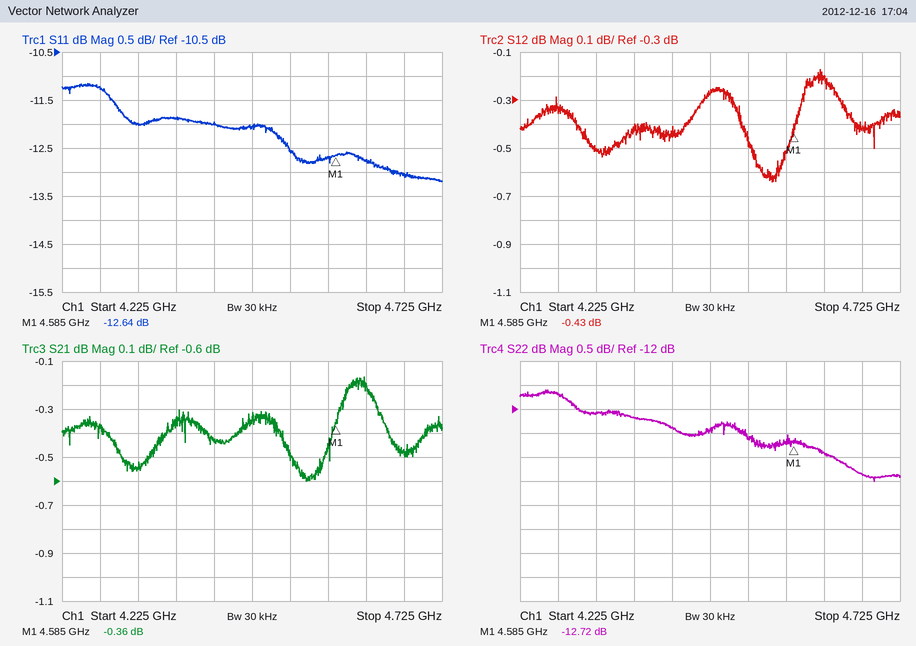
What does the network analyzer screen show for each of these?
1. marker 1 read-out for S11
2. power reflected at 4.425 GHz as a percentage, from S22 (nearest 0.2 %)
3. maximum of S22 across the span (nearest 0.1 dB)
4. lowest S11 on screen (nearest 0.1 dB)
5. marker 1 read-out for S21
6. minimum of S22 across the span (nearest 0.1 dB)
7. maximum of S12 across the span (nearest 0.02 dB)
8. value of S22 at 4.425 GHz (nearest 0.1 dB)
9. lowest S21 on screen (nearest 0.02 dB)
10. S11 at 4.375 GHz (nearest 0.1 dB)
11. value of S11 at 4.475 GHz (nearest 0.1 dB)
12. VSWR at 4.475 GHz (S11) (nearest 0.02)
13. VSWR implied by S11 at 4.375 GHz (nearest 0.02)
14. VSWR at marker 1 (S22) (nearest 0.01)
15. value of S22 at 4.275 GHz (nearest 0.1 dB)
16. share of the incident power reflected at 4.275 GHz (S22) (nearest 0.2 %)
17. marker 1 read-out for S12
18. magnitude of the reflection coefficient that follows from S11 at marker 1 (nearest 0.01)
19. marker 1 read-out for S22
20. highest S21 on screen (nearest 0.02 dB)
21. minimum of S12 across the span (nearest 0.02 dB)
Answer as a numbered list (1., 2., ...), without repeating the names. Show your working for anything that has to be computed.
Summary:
1. -12.64 dB
2. 10^(-12.4/10) ≈ 5.8 %
3. -11.6 dB
4. -13.2 dB
5. -0.36 dB
6. -13.5 dB
7. -0.18 dB
8. -12.4 dB
9. -0.60 dB
10. -11.9 dB
11. -12.1 dB
12. |Γ| = 10^(-12.1/20) = 0.2483; VSWR = (1 + 0.2483)/(1 − 0.2483) ≈ 1.66
13. |Γ| = 10^(-11.9/20) = 0.2541; VSWR = (1 + 0.2541)/(1 − 0.2541) ≈ 1.68
14. (1 + 0.2312)/(1 − 0.2312) ≈ 1.60
15. -11.7 dB
16. 10^(-11.7/10) ≈ 6.8 %
17. -0.43 dB
18. 10^(-12.64/20) ≈ 0.23
19. -12.72 dB
20. -0.16 dB
21. -0.64 dB
